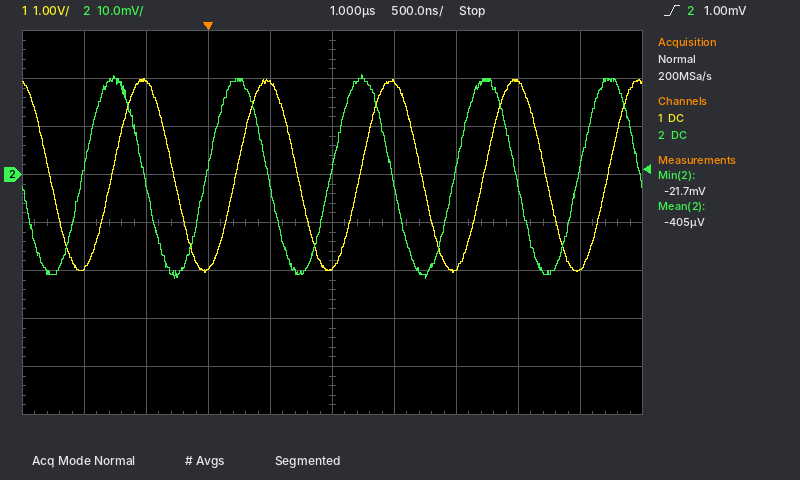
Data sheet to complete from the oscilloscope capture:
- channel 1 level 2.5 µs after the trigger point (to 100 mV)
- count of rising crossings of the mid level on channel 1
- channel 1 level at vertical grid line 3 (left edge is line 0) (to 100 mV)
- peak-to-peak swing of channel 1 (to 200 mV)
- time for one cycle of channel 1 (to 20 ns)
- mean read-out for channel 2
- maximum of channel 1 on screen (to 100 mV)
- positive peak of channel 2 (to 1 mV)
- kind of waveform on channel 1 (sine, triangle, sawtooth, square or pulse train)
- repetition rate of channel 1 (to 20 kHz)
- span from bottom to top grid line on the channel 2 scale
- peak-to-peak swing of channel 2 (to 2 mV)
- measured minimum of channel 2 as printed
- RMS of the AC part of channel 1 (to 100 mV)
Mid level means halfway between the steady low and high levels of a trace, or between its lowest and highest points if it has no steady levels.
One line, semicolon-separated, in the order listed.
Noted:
1.9 V; 5; -2.0 V; 4.0 V; 1.00 µs; -405 µV; 2.0 V; 21 mV; sine; 1.00 MHz; 80 mV; 42 mV; -21.7 mV; 1.4 V
